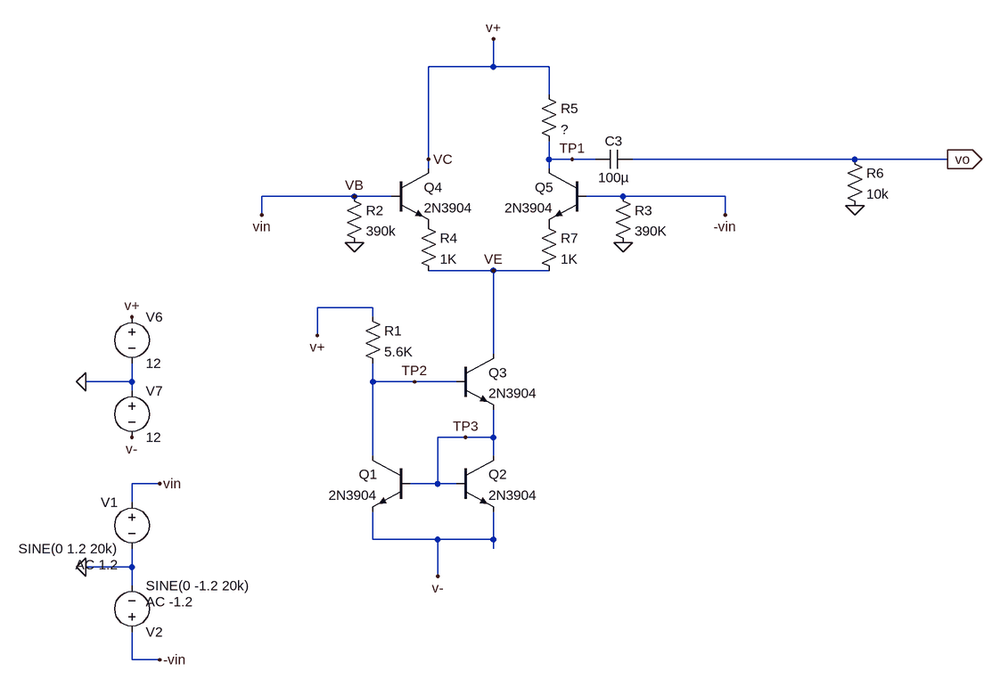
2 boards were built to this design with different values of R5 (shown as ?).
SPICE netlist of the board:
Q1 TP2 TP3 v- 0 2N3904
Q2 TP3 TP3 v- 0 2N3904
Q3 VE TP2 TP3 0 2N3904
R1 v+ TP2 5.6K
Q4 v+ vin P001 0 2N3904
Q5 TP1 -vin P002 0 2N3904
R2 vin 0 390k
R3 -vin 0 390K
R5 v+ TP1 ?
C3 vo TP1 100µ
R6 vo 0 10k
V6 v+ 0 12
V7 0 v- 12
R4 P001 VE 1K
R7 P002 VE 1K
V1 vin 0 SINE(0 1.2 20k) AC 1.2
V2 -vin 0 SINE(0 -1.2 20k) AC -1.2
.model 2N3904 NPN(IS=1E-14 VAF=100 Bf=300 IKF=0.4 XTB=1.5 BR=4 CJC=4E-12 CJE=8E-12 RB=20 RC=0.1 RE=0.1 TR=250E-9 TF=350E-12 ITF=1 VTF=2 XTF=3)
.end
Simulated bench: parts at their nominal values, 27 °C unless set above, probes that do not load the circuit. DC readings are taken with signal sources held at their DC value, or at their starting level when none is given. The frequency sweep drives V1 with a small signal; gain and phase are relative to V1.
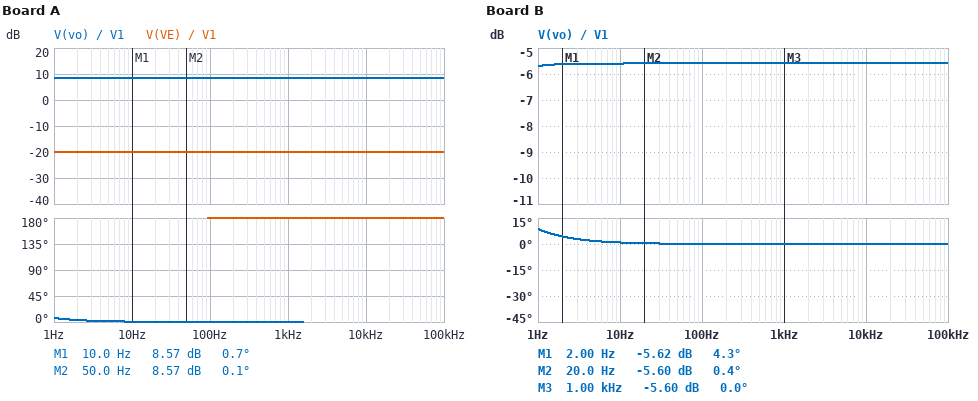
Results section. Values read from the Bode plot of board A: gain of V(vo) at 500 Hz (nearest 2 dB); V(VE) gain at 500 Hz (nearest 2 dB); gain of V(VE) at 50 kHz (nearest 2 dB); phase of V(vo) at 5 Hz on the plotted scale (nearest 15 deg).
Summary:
8 dB
-20 dB
-20 dB
0 deg
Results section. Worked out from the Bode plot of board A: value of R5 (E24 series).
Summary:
3.3 kΩ
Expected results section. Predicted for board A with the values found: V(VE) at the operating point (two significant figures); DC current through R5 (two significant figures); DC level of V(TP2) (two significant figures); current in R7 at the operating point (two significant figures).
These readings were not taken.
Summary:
-2.7 V
2.0 mA
-11 V
2.0 mA
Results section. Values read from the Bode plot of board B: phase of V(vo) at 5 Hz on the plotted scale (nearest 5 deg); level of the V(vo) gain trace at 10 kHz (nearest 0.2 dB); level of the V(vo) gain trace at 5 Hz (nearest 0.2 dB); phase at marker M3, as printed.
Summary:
0 deg
-5.6 dB
-5.6 dB
0.0 deg
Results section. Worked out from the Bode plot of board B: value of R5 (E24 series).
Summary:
510 Ω
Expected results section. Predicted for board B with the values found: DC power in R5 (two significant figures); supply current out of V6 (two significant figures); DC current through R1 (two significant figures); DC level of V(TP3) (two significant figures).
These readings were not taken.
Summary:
2.0 mW
8.0 mA
4.0 mA
-11 V
